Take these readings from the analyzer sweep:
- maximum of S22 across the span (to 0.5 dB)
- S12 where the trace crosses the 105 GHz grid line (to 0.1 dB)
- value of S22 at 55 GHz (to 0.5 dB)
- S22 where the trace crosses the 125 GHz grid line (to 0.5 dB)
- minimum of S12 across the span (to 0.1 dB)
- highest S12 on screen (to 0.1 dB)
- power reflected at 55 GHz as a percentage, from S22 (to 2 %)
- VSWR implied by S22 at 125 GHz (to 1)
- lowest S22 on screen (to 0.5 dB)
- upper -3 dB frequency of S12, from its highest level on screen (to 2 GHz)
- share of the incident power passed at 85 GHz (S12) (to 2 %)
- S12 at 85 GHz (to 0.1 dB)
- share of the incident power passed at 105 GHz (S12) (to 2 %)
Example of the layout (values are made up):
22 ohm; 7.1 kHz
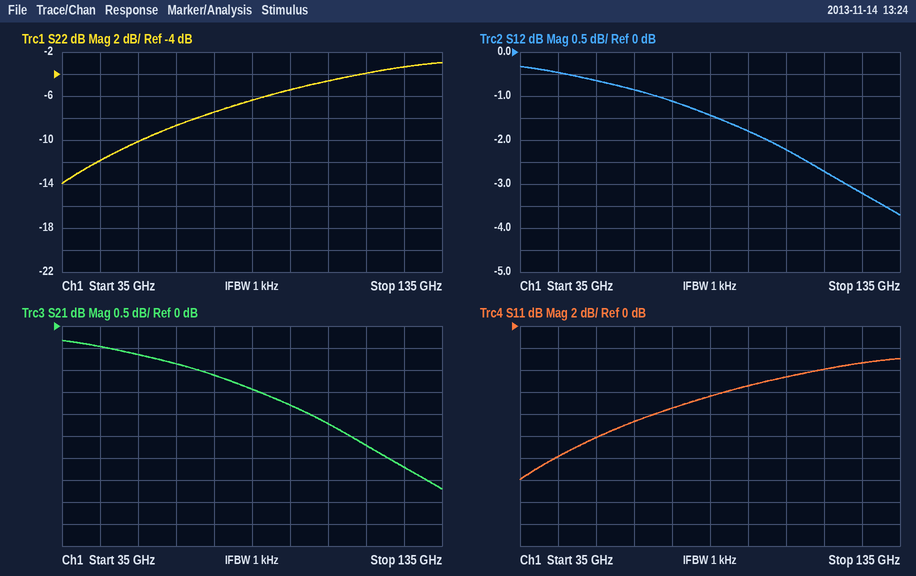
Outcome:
-3.0 dB; -2.2 dB; -10.0 dB; -3.5 dB; -3.7 dB; -0.3 dB; 10 %; 5; -14.0 dB; 128 GHz; 72 %; -1.4 dB; 60 %
